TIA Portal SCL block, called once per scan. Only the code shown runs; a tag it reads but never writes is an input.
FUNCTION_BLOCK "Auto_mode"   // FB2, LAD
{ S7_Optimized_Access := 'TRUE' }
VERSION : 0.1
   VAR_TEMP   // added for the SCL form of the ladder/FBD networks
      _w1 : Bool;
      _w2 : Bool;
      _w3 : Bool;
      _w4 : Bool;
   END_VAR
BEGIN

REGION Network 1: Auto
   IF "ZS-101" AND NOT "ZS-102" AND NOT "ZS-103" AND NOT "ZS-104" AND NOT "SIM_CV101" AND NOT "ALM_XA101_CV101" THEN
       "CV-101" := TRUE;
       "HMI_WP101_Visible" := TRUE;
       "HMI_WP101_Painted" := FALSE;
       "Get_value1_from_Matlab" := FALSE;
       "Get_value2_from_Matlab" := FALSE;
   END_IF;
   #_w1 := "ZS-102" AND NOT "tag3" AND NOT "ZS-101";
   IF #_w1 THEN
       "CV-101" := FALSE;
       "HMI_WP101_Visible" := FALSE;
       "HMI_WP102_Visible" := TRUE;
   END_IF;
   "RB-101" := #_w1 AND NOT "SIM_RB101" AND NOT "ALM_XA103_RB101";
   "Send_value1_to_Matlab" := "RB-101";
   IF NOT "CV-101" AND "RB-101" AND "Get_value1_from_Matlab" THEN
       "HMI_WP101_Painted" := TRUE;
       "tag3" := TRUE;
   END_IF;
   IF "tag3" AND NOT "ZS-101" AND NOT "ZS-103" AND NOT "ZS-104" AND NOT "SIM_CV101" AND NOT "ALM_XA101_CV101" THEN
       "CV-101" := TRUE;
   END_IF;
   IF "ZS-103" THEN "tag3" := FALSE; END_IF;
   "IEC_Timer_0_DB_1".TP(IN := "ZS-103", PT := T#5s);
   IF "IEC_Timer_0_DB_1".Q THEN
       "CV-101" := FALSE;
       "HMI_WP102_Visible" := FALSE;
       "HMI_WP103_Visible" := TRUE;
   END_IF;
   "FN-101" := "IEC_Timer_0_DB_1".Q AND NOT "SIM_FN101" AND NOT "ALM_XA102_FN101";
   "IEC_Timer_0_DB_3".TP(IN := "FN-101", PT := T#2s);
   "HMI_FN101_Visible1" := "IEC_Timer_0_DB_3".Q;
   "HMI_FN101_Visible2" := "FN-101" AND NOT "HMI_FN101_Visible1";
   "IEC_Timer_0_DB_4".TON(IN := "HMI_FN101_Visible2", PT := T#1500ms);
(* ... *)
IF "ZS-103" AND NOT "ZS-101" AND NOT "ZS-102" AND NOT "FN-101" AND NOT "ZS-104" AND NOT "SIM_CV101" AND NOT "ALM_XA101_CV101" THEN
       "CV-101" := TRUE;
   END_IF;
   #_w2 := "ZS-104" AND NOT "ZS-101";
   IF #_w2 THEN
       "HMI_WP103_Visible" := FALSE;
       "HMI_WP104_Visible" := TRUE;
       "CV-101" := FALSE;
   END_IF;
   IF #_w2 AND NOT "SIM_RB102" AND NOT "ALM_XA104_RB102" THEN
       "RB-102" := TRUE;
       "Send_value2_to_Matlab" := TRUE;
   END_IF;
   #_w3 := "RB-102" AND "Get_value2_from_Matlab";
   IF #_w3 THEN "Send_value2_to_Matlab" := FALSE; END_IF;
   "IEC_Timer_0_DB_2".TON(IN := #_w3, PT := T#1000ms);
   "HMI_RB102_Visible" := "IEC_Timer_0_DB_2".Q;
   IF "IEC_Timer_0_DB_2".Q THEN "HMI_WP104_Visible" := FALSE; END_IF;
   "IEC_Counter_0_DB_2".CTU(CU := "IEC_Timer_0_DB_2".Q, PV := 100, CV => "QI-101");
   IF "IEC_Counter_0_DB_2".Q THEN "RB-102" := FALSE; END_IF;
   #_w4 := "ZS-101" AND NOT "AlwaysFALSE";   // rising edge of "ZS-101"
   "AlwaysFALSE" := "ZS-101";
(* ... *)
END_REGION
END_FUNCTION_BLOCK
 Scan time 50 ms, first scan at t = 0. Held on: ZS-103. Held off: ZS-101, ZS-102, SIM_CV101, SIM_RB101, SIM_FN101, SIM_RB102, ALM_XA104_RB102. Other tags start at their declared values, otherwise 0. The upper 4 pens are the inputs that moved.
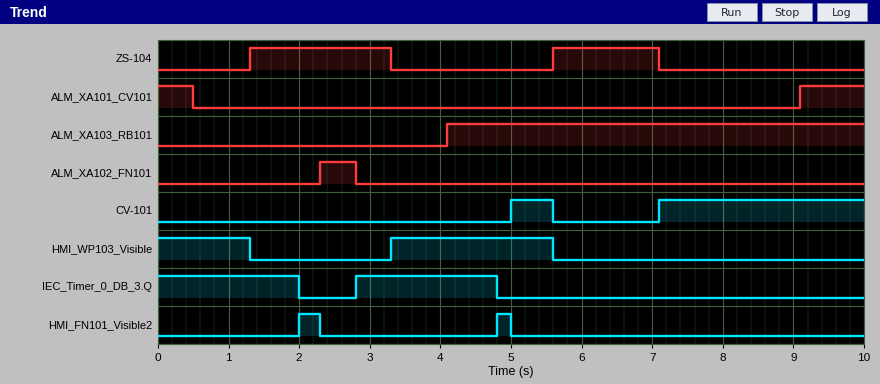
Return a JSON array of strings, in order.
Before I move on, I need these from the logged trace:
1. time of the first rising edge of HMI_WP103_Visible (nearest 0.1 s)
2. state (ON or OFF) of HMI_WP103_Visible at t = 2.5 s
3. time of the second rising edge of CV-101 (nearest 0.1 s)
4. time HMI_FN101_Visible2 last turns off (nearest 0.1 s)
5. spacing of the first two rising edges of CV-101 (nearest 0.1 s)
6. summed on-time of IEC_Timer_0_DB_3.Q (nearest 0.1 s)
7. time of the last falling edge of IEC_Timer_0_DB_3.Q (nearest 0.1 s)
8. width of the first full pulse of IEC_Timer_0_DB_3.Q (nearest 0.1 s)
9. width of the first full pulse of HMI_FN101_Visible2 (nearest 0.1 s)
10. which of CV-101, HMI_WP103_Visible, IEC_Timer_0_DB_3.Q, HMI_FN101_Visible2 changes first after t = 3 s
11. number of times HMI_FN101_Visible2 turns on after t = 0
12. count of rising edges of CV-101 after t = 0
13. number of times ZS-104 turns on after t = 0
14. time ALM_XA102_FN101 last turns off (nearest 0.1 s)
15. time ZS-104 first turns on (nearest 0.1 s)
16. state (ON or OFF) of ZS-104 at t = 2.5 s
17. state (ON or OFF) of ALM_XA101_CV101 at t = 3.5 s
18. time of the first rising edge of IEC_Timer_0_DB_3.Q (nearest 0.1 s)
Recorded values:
["3.3 s", "OFF", "7.1 s", "5.0 s", "2.1 s", "4.0 s", "4.8 s", "2.0 s", "0.3 s", "HMI_WP103_Visible", "2", "2", "2", "2.8 s", "1.3 s", "ON", "OFF", "2.8 s"]
